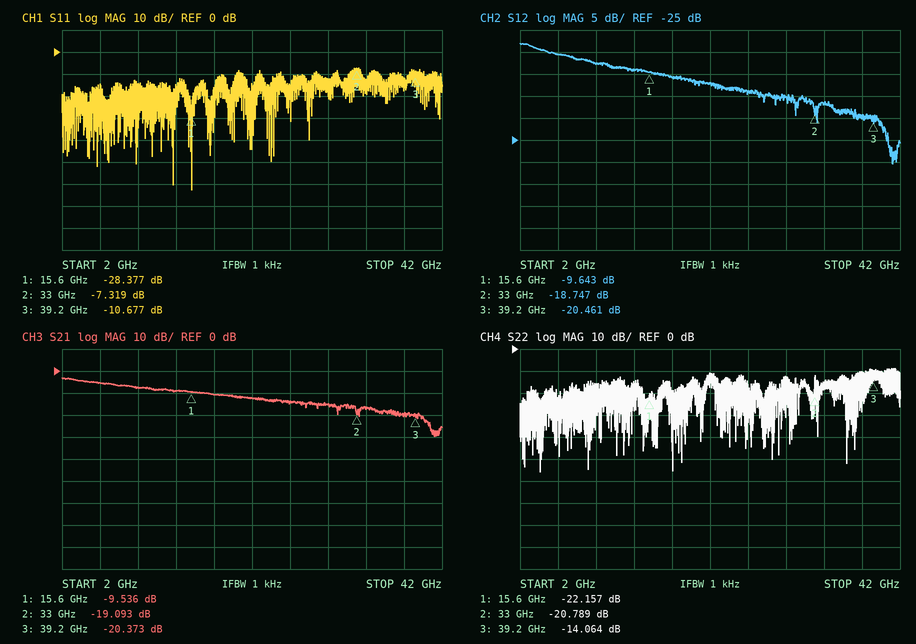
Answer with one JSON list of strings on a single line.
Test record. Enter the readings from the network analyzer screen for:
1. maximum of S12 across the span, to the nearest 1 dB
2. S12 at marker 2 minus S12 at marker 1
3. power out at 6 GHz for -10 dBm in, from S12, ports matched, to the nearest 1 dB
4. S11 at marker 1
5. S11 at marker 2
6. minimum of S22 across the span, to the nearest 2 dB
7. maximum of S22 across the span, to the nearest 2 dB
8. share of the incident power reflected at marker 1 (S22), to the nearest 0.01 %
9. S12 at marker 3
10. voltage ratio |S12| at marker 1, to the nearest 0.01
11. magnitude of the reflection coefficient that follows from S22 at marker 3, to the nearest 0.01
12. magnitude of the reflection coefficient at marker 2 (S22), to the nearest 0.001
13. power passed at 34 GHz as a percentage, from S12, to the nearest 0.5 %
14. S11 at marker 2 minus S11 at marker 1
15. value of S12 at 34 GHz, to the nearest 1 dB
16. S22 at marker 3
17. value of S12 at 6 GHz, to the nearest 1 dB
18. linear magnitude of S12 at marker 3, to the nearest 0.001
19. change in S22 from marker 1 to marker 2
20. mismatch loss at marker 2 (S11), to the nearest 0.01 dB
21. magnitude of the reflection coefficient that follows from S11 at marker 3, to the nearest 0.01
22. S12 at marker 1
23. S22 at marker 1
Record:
["-3 dB", "-9.104 dB", "-16 dBm", "-28.377 dB", "-7.319 dB", "-56 dB", "-8 dB", "0.61 %", "-20.461 dB", "0.33", "0.20", "0.091", "2.0 %", "21.058 dB", "-17 dB", "-14.064 dB", "-6 dB", "0.095", "1.368 dB", "0.89 dB", "0.29", "-9.643 dB", "-22.157 dB"]
